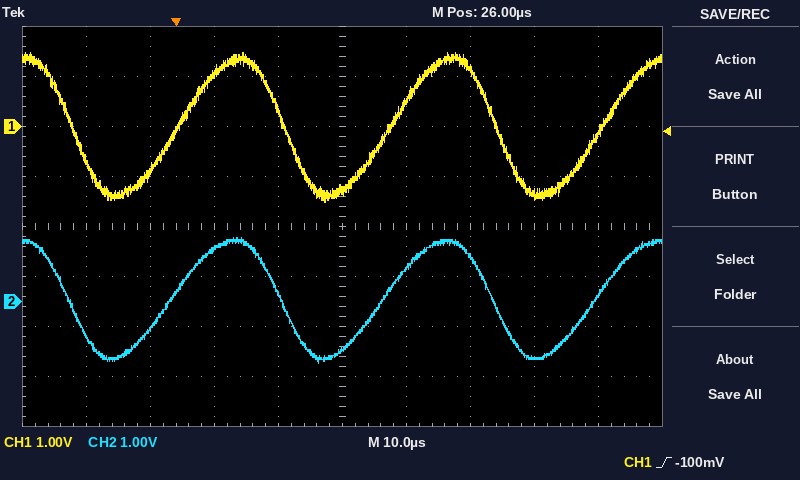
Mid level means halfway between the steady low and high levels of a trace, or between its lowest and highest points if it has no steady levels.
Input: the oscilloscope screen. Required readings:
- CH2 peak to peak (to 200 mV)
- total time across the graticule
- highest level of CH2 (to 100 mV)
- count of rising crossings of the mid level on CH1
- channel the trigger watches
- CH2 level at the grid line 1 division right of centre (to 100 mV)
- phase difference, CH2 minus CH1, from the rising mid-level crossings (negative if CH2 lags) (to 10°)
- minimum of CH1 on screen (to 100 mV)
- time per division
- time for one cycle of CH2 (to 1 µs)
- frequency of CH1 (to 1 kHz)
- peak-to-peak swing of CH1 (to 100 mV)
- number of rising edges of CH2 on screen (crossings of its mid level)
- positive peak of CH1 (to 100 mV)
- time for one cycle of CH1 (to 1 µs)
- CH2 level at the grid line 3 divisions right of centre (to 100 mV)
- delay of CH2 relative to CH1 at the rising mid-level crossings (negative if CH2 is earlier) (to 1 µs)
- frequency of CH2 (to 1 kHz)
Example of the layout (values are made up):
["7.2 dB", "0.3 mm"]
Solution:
["2.6 V", "100 µs", "1.3 V", "3", "CH1", "700 mV", "+10°", "-1.5 V", "10 µs", "33 µs", "30 kHz", "3.0 V", "3", "1.5 V", "33 µs", "-1.1 V", "-1 µs", "30 kHz"]
